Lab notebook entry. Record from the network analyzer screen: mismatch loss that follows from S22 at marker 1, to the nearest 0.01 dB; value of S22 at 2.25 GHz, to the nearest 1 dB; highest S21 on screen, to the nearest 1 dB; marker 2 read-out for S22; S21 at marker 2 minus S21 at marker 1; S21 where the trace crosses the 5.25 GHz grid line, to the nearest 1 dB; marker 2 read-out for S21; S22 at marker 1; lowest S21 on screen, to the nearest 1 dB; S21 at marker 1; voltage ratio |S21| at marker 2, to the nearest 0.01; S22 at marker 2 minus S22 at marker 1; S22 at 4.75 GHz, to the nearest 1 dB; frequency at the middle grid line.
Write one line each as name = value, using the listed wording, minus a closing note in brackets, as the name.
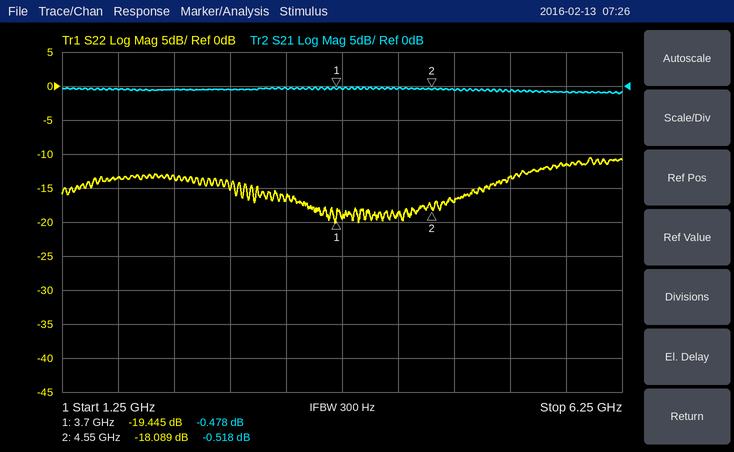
mismatch loss that follows from S22 at marker 1, to the nearest 0.01 dB = 0.05 dB
value of S22 at 2.25 GHz, to the nearest 1 dB = -13 dB
highest S21 on screen, to the nearest 1 dB = 0 dB
marker 2 read-out for S22 = -18.089 dB
S21 at marker 2 minus S21 at marker 1 = -0.040 dB
S21 where the trace crosses the 5.25 GHz grid line, to the nearest 1 dB = -1 dB
marker 2 read-out for S21 = -0.518 dB
S22 at marker 1 = -19.445 dB
lowest S21 on screen, to the nearest 1 dB = -1 dB
S21 at marker 1 = -0.478 dB
voltage ratio |S21| at marker 2, to the nearest 0.01 = 0.94
S22 at marker 2 minus S22 at marker 1 = 1.356 dB
S22 at 4.75 GHz, to the nearest 1 dB = -17 dB
frequency at the middle grid line = 3.75 GHz
